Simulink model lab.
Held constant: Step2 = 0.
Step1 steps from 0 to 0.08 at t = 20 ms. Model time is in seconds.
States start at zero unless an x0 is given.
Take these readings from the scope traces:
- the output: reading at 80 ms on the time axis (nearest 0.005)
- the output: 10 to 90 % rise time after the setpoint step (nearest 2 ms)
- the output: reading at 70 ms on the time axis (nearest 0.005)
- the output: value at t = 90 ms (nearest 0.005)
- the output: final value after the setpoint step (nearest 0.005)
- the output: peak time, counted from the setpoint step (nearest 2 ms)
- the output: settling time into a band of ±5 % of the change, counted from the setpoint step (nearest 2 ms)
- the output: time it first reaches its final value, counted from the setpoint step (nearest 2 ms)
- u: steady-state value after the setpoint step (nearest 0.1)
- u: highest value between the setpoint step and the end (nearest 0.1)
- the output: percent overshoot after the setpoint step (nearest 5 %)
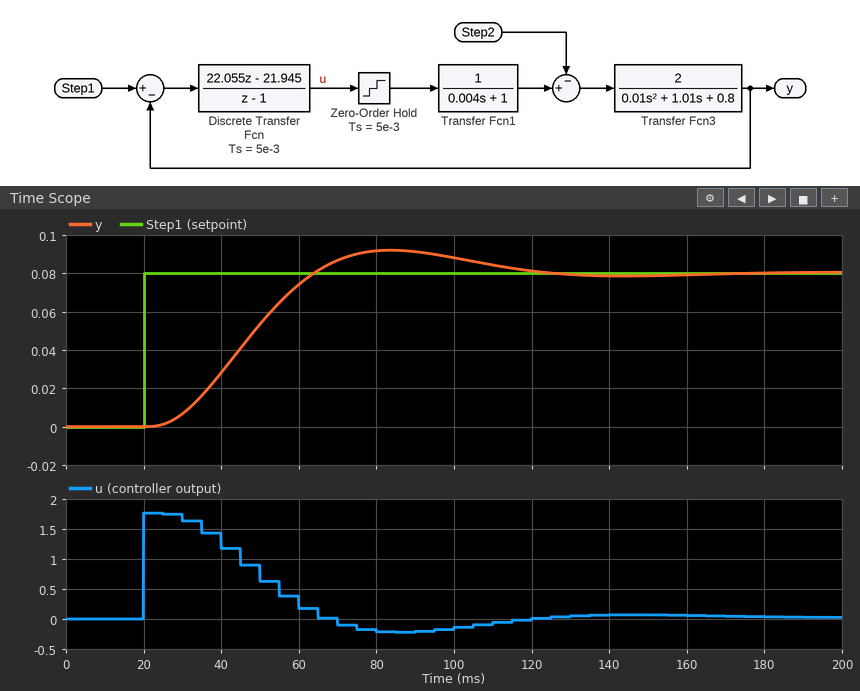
0.090
28 ms
0.085
0.090
0.080
64 ms
90 ms
44 ms
0.0
1.8
15 %
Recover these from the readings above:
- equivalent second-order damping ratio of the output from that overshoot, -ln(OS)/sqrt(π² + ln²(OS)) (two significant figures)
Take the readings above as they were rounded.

0.52
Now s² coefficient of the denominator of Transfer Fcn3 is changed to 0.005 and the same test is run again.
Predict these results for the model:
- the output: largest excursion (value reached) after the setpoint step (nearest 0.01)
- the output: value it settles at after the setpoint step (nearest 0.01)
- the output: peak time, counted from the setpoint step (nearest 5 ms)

0.08
0.08
60 ms
